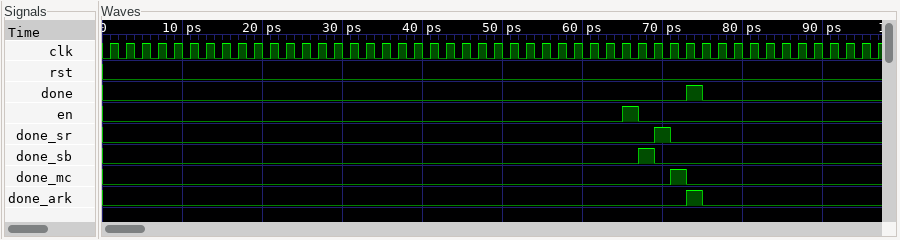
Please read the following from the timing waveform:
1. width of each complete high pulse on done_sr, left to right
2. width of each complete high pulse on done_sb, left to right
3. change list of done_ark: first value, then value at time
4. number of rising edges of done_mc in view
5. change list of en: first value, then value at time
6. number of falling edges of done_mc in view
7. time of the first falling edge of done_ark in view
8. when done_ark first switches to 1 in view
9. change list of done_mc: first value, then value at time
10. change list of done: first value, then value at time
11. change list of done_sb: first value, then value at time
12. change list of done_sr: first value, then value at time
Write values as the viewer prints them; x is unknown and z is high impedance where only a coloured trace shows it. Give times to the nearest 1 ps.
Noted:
2 ps
2 ps
0, 1 at 73 ps, 0 at 75 ps
1
0, 1 at 65 ps, 0 at 67 ps
1
75 ps
73 ps
0, 1 at 71 ps, 0 at 73 ps
0, 1 at 73 ps, 0 at 75 ps
0, 1 at 67 ps, 0 at 69 ps
0, 1 at 69 ps, 0 at 71 ps
